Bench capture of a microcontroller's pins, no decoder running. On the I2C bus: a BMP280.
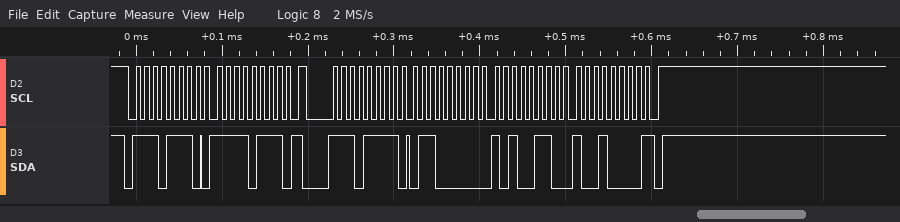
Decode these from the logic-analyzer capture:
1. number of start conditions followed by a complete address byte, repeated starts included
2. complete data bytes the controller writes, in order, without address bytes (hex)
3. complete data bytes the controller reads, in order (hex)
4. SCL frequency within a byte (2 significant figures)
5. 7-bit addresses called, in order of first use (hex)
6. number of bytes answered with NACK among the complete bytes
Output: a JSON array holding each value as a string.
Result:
["2", "F7", "60 A6 90", "100 kHz", "0x77", "1"]
